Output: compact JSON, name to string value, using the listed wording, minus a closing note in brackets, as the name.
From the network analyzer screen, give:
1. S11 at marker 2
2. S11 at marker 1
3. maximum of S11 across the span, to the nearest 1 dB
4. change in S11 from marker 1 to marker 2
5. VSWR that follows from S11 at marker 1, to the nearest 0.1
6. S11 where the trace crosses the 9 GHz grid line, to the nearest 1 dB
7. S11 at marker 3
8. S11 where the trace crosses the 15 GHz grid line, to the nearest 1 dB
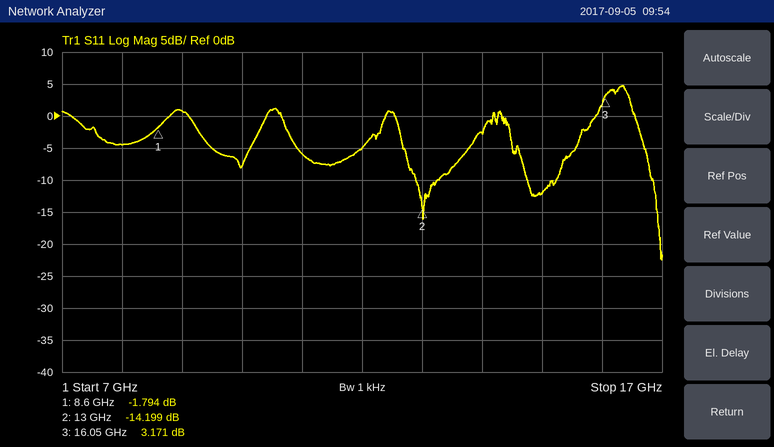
{"S11 at marker 2": "-14.199 dB", "S11 at marker 1": "-1.794 dB", "maximum of S11 across the span, to the nearest 1 dB": "5 dB", "change in S11 from marker 1 to marker 2": "-12.405 dB", "VSWR that follows from S11 at marker 1, to the nearest 0.1": "9.7", "S11 where the trace crosses the 9 GHz grid line, to the nearest 1 dB": "1 dB", "S11 at marker 3": "3.171 dB", "S11 where the trace crosses the 15 GHz grid line, to the nearest 1 dB": "-12 dB"}
